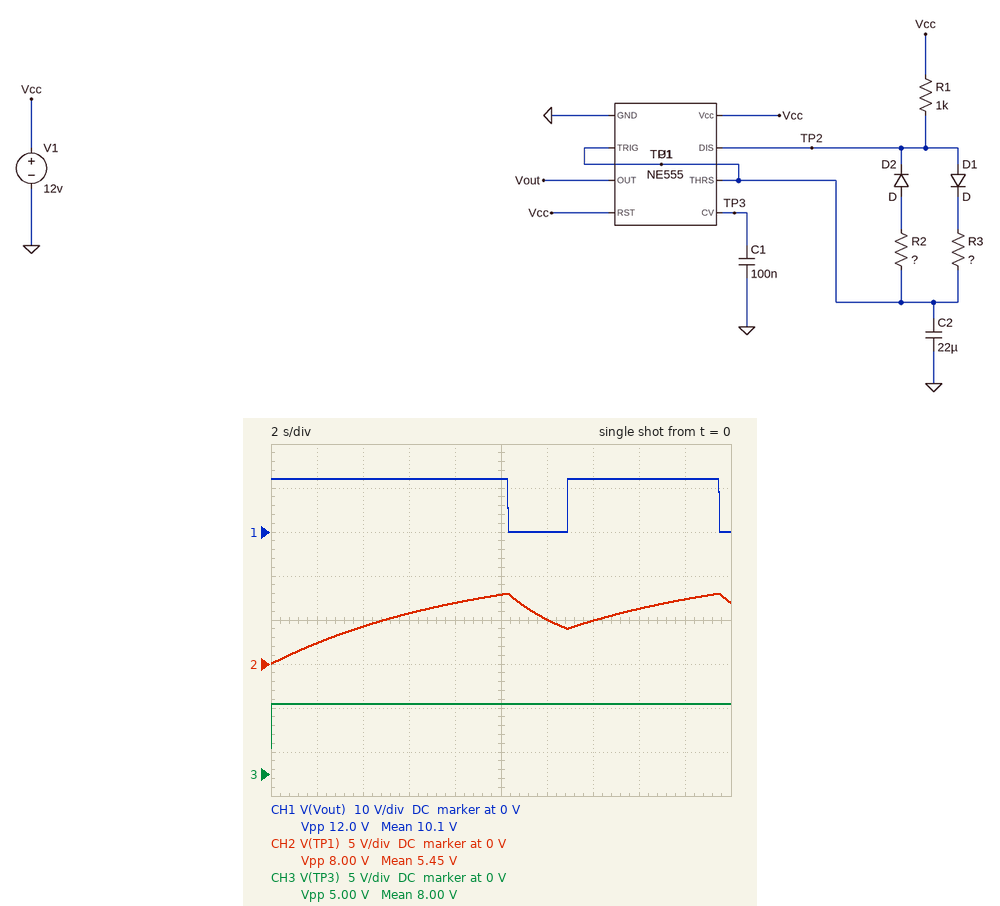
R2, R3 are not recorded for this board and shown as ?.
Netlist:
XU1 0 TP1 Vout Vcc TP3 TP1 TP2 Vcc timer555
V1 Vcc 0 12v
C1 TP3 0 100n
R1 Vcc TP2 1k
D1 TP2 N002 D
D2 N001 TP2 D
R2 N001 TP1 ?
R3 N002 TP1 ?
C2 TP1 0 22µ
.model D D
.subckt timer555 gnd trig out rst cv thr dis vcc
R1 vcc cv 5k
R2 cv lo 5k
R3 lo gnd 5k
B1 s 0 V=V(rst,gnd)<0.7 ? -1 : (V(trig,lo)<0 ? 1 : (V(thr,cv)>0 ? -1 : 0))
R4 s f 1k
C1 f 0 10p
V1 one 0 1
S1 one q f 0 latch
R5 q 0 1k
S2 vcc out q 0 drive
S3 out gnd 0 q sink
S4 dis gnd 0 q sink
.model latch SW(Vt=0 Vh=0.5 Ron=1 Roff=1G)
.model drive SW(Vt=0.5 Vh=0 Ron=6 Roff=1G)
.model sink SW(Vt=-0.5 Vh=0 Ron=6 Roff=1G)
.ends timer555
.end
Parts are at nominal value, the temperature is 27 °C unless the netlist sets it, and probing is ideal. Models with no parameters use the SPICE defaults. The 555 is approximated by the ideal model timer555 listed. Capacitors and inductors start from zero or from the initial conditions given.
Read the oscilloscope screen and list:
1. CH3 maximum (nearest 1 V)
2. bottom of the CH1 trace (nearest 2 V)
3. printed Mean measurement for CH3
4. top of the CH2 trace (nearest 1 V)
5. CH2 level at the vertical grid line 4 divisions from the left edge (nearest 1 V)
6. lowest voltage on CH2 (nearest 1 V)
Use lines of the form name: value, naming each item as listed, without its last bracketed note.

CH3 maximum: 8 V
bottom of the CH1 trace: 0 V
printed Mean measurement for CH3: 8.00 V
top of the CH2 trace: 8 V
CH2 level at the vertical grid line 4 divisions from the left edge: 7 V
lowest voltage on CH2: 0 V
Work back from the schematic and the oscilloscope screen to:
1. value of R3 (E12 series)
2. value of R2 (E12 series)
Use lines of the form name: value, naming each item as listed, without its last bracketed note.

value of R3: 390 kΩ
value of R2: 150 kΩ
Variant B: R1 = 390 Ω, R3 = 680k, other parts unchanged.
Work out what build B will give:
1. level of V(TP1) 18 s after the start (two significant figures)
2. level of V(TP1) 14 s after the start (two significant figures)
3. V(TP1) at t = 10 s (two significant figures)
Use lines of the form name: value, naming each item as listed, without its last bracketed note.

level of V(TP1) 18 s after the start: 7.8 V
level of V(TP1) 14 s after the start: 7.0 V
V(TP1) at t = 10 s: 5.6 V
